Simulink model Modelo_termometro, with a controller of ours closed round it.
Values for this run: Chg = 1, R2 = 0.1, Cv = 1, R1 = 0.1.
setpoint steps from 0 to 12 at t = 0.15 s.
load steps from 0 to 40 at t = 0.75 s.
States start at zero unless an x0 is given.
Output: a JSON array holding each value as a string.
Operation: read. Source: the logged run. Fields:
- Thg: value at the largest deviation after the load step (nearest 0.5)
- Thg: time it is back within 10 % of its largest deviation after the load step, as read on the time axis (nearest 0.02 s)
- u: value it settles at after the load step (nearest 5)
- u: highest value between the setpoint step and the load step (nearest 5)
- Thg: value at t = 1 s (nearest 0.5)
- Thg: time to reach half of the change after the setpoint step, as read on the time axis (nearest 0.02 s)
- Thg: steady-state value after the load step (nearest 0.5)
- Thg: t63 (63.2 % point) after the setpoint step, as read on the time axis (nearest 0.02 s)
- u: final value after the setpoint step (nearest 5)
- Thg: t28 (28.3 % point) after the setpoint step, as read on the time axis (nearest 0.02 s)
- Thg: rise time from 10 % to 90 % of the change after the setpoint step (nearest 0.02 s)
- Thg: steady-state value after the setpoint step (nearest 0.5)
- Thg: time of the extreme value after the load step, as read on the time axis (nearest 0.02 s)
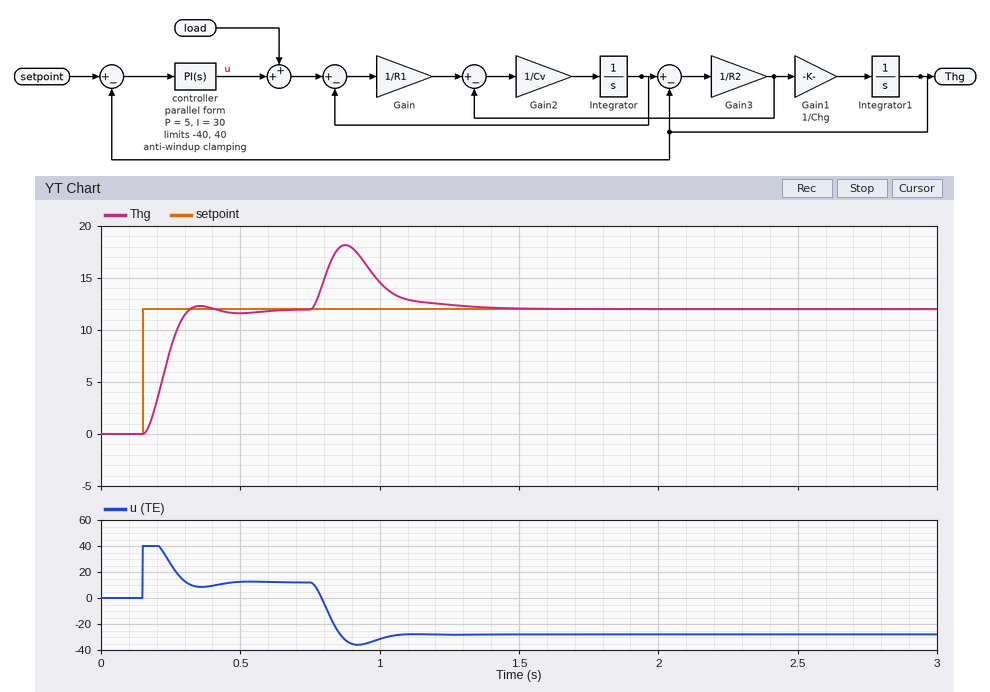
["18.0", "1.18 s", "-30", "40", "14.5", "0.22 s", "12.0", "0.24 s", "10", "0.20 s", "0.10 s", "12.0", "0.88 s"]
